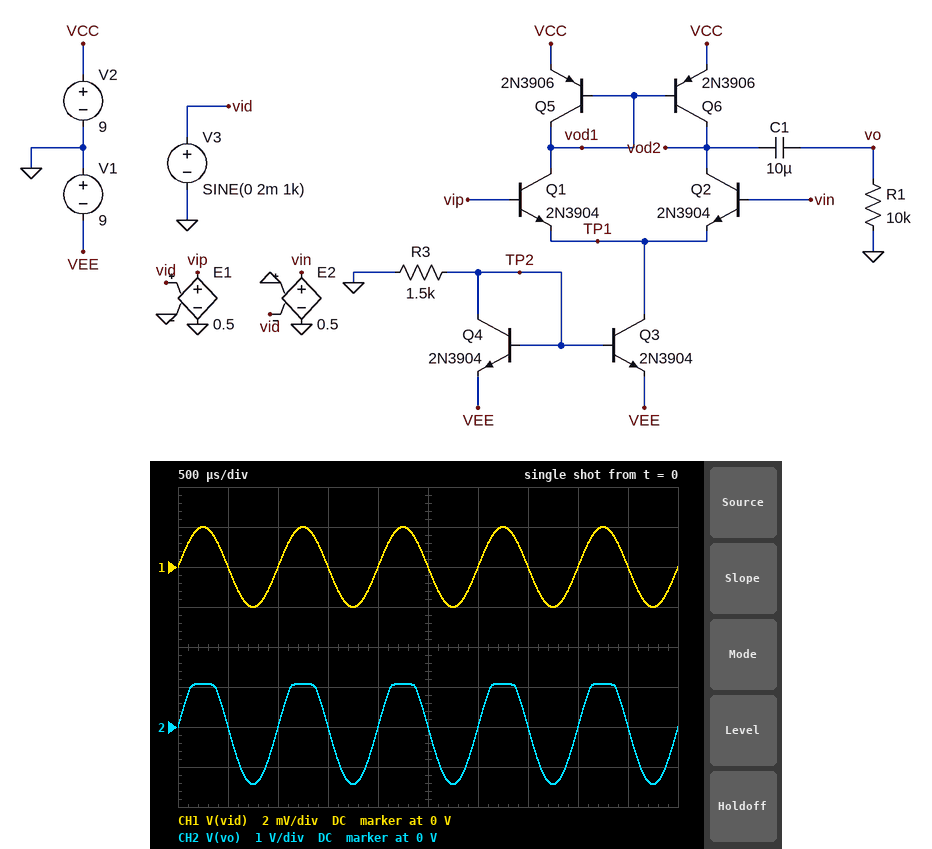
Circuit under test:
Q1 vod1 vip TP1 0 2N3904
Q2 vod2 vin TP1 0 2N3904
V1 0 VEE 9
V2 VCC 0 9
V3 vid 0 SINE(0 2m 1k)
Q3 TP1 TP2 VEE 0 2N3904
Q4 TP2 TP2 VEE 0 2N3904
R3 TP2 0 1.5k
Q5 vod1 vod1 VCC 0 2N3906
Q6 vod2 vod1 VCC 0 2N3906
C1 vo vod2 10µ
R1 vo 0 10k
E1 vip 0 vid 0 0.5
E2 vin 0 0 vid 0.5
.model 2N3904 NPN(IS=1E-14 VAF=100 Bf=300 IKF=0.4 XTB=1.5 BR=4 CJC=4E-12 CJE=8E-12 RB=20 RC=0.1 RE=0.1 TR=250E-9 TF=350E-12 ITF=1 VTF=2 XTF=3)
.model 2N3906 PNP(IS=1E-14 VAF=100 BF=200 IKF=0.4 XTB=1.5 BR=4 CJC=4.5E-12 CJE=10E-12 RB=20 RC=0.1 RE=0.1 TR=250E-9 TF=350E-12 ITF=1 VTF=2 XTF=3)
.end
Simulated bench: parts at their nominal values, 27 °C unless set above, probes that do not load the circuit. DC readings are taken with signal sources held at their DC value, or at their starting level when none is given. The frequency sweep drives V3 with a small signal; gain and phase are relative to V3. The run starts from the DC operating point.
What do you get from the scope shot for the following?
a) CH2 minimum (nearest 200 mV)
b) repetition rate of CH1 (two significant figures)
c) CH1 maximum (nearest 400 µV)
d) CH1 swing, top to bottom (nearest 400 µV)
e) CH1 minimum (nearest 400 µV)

-1.4 V
1.0 kHz
2.0 mV
4.0 mV
-2.0 mV
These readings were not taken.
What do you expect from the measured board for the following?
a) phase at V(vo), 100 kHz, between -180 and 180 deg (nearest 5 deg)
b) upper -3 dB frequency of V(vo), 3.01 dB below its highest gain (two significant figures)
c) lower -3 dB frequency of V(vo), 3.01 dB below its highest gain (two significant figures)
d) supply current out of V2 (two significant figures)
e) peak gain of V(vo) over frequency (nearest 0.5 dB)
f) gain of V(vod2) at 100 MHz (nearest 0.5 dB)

-5 deg
1.1 MHz
570 mHz
5.9 mA
57.0 dB
18.0 dB
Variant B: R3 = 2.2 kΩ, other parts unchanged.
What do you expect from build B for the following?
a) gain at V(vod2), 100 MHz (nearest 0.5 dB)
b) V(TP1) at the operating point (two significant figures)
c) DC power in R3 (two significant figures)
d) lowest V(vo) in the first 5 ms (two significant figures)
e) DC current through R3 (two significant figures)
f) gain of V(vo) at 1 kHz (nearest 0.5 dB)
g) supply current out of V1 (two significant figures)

16.5 dB
-670 mV
31 mW
-1.1 V
3.8 mA
55.0 dB
7.8 mA
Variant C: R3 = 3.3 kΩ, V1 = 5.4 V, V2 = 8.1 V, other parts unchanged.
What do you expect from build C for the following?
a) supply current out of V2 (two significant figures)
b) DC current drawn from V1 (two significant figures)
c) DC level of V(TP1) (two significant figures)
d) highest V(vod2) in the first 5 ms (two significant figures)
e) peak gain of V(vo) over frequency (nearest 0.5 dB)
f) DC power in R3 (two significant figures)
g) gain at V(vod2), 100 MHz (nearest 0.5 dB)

1.5 mA
2.9 mA
-650 mV
7.4 V
48.0 dB
6.8 mW
10.5 dB
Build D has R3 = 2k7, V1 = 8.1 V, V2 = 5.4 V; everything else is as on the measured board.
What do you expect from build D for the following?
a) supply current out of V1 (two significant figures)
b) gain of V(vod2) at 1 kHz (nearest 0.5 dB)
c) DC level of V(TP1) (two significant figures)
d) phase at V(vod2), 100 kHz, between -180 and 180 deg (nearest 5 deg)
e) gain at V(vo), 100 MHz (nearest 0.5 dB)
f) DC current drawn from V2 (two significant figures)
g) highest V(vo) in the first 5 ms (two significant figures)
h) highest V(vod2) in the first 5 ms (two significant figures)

5.7 mA
52.5 dB
-660 mV
-5 deg
14.5 dB
2.9 mA
860 mV
5.1 V
